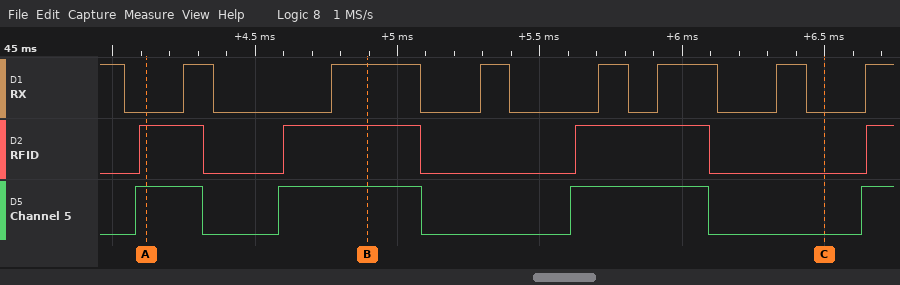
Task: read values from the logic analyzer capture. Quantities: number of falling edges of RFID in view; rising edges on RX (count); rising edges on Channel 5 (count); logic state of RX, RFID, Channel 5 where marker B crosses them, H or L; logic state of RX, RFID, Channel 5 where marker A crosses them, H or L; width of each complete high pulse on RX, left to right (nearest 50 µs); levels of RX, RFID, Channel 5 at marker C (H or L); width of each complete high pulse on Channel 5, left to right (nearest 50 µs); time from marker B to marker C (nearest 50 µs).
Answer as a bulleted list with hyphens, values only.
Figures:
- 3
- 7
- 4
- RX=H, RFID=H, Channel 5=H
- RX=L, RFID=H, Channel 5=H
- 100 µs, 300 µs, 100 µs, 100 µs, 200 µs, 100 µs
- RX=L, RFID=L, Channel 5=L
- 250 µs, 500 µs, 500 µs
- 1600 µs
